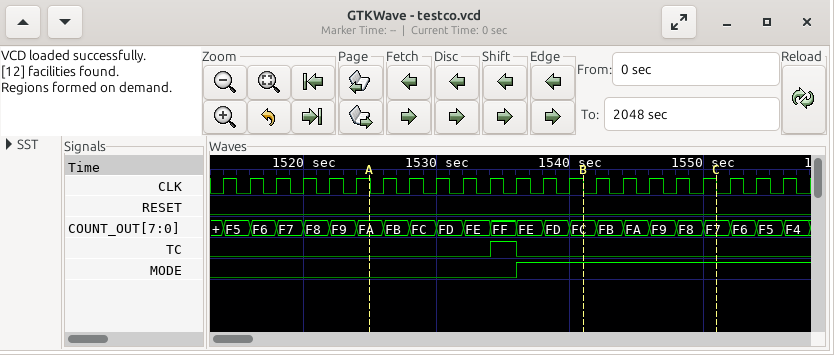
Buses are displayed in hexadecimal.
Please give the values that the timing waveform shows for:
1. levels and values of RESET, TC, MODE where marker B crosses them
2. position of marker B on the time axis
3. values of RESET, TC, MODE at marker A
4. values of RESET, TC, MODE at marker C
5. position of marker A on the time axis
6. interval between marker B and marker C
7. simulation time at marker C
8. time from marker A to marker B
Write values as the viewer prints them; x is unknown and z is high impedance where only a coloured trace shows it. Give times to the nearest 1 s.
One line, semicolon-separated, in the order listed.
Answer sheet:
RESET=0, TC=0, MODE=1; 1541 s; RESET=0, TC=0, MODE=0; RESET=0, TC=0, MODE=1; 1525 s; 10 s; 1551 s; 16 s
